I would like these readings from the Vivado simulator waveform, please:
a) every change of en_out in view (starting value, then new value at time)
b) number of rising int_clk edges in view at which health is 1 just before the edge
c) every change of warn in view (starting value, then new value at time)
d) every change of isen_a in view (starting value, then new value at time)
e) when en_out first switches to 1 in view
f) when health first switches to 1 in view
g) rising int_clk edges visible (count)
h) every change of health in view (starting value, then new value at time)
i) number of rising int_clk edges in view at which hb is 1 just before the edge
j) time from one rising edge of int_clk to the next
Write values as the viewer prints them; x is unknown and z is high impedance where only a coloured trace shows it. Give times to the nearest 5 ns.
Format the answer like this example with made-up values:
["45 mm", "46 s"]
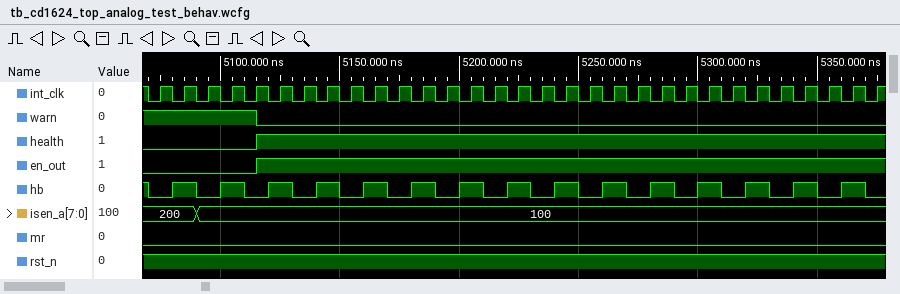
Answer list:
["0, 1 at 5115 ns", "26", "1, 0 at 5115 ns", "200, 100 at 5090 ns", "5115 ns", "5115 ns", "31", "0, 1 at 5115 ns", "15", "10 ns"]
